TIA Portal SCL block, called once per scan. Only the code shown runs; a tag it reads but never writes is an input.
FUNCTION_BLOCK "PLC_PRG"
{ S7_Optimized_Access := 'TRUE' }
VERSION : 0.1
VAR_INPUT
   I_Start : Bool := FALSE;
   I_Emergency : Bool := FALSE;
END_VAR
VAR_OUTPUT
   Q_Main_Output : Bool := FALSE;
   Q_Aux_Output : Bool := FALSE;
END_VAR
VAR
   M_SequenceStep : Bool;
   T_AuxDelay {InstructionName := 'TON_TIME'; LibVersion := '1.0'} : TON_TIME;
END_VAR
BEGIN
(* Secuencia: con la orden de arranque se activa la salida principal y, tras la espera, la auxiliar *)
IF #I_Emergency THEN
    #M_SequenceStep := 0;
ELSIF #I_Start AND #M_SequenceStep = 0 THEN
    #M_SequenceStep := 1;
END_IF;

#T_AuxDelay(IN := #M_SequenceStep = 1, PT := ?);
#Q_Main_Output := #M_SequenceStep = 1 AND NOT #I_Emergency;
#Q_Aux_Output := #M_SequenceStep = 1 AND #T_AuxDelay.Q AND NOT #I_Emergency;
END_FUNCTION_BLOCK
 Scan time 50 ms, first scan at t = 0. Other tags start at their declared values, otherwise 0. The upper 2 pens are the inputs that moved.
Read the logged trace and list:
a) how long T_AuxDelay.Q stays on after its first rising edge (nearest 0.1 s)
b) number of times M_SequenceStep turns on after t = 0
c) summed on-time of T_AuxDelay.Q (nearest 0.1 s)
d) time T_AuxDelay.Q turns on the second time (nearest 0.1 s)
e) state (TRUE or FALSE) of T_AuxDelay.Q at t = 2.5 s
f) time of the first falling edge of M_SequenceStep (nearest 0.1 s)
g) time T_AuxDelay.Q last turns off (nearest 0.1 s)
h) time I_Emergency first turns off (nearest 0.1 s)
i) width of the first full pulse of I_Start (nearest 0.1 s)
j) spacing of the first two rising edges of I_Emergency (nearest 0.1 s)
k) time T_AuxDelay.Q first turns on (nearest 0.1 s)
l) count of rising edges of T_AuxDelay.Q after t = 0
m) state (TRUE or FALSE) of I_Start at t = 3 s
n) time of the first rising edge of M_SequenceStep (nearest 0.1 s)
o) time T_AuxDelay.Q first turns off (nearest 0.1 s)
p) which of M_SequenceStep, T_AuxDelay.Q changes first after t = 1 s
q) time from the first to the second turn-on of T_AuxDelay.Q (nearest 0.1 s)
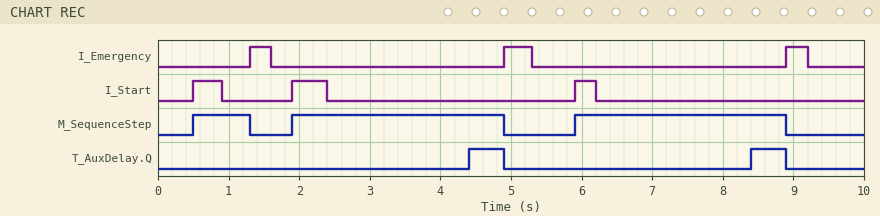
0.5 s
3
1.0 s
8.4 s
FALSE
1.3 s
8.9 s
1.6 s
0.4 s
3.6 s
4.4 s
2
FALSE
0.5 s
4.9 s
M_SequenceStep
4.0 s
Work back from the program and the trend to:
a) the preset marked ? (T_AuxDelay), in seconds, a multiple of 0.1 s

2.5 s
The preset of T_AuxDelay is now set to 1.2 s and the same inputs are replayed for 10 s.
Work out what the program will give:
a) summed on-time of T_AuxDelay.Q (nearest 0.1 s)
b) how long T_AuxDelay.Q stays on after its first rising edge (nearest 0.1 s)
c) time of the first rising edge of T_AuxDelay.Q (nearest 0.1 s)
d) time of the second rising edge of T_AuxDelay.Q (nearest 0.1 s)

3.6 s
1.8 s
3.1 s
7.1 s
